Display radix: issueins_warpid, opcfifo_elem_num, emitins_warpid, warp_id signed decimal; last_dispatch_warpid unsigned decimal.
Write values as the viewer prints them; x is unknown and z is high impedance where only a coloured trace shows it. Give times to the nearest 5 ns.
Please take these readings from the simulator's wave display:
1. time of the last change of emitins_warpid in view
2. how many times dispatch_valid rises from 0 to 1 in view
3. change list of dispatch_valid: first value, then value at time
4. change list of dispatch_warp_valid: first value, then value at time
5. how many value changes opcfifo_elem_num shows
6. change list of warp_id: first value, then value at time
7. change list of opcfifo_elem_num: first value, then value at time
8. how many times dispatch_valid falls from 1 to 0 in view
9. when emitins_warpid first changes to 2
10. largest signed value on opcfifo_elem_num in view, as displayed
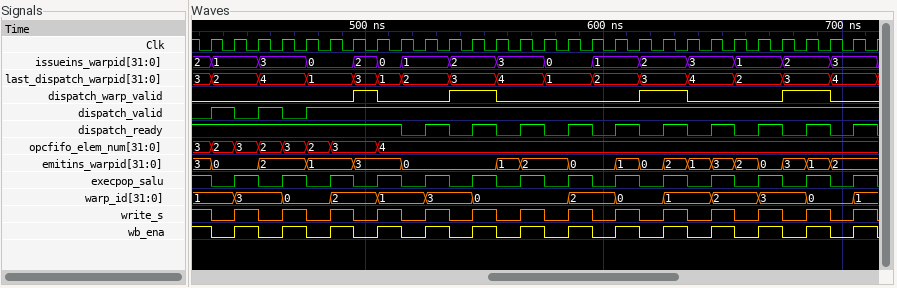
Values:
695 ns
3
0, 1 at 435 ns, 0 at 445 ns, 1 at 455 ns, 0 at 465 ns, 1 at 475 ns
0, 1 at 495 ns, 0 at 505 ns, 1 at 535 ns, 0 at 555 ns, 1 at 615 ns, 0 at 635 ns, 1 at 675 ns, 0 at 695 ns
7
1, 3 at 445 ns, 0 at 465 ns, 2 at 485 ns, 1 at 505 ns, 3 at 525 ns, 0 at 545 ns, 2 at 585 ns, 0 at 605 ns, 1 at 625 ns, 2 at 645 ns, 3 at 665 ns, 0 at 685 ns, 1 at 705 ns
3, 2 at 435 ns, 3 at 445 ns, 2 at 455 ns, 3 at 465 ns, 2 at 475 ns, 3 at 485 ns, 4 at 505 ns
2
455 ns
4
